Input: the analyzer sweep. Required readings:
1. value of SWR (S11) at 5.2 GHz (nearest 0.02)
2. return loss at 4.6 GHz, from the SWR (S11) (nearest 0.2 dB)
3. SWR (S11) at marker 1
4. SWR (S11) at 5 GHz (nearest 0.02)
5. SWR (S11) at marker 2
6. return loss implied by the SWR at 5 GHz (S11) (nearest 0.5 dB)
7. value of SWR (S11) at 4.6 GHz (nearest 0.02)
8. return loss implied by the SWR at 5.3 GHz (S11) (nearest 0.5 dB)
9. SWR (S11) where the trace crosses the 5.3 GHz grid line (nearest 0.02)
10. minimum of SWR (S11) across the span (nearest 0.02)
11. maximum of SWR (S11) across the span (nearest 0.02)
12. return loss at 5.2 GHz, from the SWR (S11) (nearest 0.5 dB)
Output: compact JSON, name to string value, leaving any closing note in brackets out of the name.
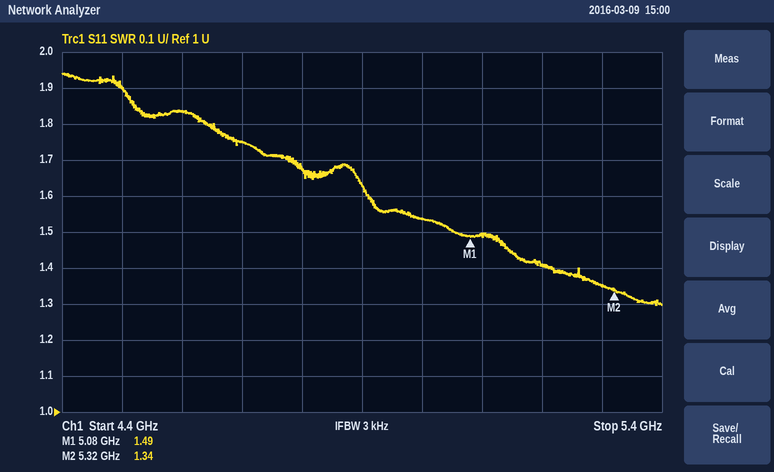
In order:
{"value of SWR (S11) at 5.2 GHz": "1.40", "return loss at 4.6 GHz, from the SWR (S11)": "10.6 dB", "SWR (S11) at marker 1": "1.49", "SWR (S11) at 5 GHz": "1.54", "SWR (S11) at marker 2": "1.34", "return loss implied by the SWR at 5 GHz (S11)": "13.5 dB", "value of SWR (S11) at 4.6 GHz": "1.84", "return loss implied by the SWR at 5.3 GHz (S11)": "16.5 dB", "SWR (S11) where the trace crosses the 5.3 GHz grid line": "1.36", "minimum of SWR (S11) across the span": "1.30", "maximum of SWR (S11) across the span": "1.94", "return loss at 5.2 GHz, from the SWR (S11)": "15.5 dB"}
